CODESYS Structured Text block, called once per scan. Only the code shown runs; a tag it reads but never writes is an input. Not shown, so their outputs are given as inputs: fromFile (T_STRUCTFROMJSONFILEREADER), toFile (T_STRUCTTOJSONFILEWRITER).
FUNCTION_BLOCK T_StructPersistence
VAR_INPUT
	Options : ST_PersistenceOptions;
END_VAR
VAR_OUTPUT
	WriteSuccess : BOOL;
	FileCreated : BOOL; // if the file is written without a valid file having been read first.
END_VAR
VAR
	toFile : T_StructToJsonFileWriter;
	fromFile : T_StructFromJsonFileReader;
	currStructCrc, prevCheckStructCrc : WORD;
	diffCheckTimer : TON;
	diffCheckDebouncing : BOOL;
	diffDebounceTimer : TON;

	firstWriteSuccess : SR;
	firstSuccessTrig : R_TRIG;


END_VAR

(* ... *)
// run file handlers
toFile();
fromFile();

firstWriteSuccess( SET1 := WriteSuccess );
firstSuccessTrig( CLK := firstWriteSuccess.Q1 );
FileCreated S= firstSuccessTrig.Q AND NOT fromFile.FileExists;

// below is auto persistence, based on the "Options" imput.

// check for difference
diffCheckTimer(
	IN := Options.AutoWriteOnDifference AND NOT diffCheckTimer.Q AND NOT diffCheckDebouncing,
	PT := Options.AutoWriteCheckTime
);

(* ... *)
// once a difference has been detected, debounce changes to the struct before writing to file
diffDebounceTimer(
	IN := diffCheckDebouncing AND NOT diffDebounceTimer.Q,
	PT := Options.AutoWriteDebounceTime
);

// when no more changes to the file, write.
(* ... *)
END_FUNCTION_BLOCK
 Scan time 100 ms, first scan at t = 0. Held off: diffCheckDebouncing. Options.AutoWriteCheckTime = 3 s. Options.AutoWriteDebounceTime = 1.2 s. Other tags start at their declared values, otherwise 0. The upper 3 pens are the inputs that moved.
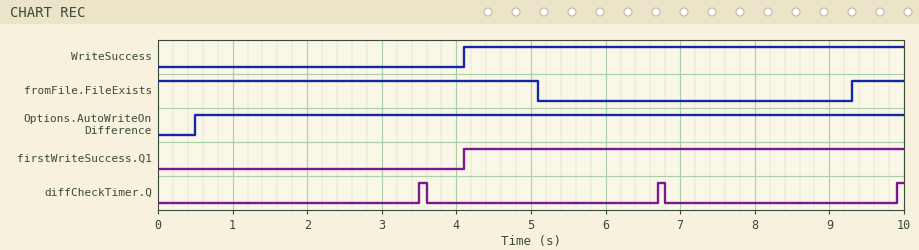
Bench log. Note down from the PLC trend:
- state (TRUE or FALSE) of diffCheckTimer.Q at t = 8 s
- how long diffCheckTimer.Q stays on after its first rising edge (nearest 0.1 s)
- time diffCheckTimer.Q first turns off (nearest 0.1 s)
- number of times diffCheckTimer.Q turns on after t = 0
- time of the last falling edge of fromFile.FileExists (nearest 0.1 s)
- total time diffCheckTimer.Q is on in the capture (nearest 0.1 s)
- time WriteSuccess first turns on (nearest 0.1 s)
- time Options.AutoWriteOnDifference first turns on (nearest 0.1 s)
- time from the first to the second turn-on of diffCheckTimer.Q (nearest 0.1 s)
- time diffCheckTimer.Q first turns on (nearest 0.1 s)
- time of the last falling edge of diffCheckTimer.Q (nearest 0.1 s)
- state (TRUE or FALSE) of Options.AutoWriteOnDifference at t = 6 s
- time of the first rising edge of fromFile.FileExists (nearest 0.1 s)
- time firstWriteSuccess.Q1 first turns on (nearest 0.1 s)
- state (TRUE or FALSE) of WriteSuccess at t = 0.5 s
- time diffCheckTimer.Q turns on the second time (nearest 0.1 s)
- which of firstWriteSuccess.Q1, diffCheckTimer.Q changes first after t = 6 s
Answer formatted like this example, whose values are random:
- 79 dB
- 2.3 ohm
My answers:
- FALSE
- 0.1 s
- 3.6 s
- 3
- 5.1 s
- 0.3 s
- 4.1 s
- 0.5 s
- 3.2 s
- 3.5 s
- 6.8 s
- TRUE
- 9.3 s
- 4.1 s
- FALSE
- 6.7 s
- diffCheckTimer.Q
